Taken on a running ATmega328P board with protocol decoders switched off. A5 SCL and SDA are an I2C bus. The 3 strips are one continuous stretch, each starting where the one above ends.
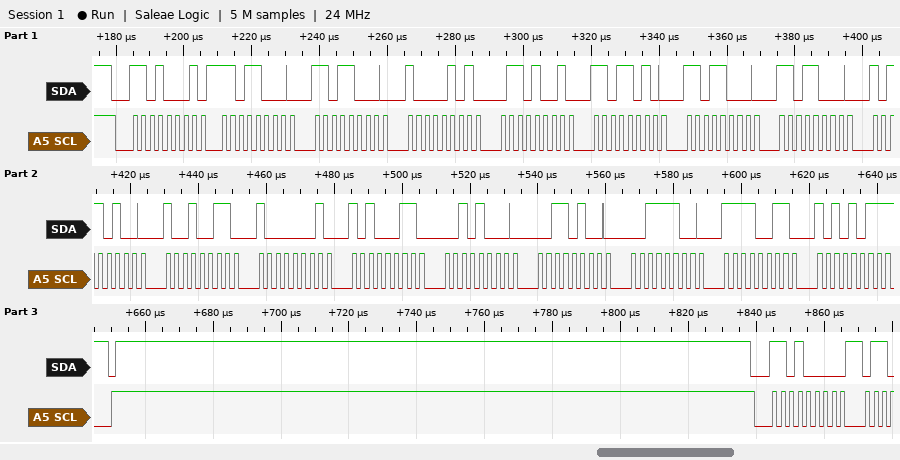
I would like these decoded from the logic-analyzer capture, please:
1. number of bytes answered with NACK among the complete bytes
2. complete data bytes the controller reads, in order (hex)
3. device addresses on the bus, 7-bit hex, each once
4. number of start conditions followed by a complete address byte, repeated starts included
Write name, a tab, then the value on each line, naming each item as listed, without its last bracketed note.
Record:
number of bytes answered with NACK among the complete bytes	1
complete data bytes the controller reads, in order	D8 D8 85 69 DA D8 D8 B4 93 81 A3 28 34 3C F3 AB
device addresses on the bus, 7-bit hex, each once	0x68
number of start conditions followed by a complete address byte, repeated starts included	2
